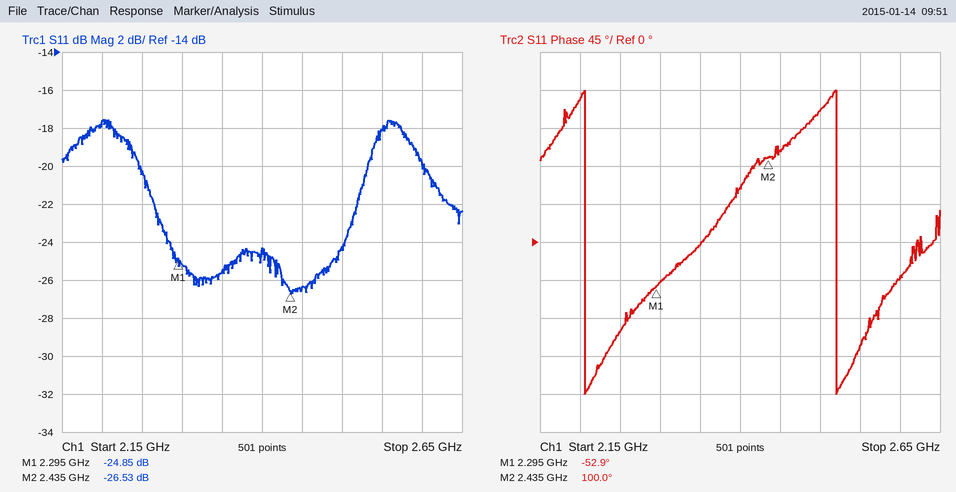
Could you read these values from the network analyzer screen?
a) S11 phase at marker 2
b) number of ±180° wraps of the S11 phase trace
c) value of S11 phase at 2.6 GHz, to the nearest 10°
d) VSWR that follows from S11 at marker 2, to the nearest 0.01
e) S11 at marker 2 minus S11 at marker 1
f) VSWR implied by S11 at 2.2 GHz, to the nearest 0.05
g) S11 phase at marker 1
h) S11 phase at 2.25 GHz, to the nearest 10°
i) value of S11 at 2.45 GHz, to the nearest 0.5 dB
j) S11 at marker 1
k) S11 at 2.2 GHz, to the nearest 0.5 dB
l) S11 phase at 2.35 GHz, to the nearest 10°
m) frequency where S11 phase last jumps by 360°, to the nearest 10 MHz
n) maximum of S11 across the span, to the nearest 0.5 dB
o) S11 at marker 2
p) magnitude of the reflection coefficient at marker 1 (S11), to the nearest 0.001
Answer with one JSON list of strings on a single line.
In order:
["100.0°", "2", "-40°", "1.10", "-1.68 dB", "1.30", "-52.9°", "-110°", "-26.5 dB", "-24.85 dB", "-17.5 dB", "0°", "2.52 GHz", "-17.5 dB", "-26.53 dB", "0.057"]
